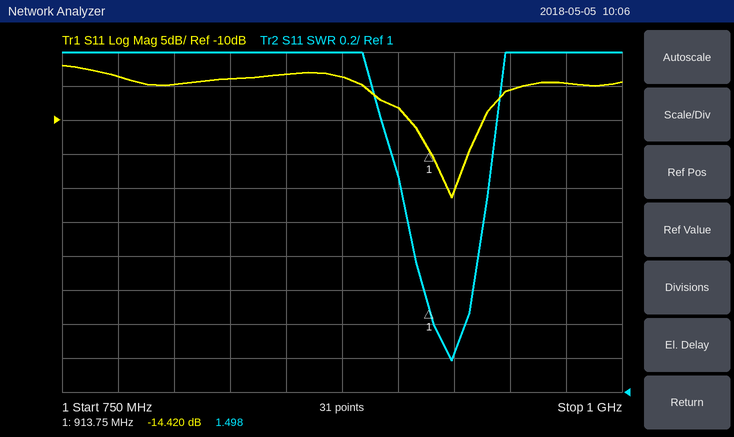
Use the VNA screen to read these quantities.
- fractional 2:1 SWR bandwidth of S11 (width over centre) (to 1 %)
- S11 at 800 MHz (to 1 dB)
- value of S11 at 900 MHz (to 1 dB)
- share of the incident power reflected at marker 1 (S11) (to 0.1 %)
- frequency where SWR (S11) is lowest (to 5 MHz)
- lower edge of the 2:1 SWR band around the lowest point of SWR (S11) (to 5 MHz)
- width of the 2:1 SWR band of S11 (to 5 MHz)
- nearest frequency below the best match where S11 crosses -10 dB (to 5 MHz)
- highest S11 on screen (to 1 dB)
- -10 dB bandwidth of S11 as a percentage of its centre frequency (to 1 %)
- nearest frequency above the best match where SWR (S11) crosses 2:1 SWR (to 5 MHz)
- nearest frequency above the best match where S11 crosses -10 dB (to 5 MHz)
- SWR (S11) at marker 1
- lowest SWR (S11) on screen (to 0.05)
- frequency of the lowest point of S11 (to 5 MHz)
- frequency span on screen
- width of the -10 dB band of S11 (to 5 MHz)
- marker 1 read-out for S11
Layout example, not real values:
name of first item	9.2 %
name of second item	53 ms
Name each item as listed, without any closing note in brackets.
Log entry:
fractional 2:1 SWR bandwidth of S11 (width over centre)	4 %
S11 at 800 MHz	-5 dB
value of S11 at 900 MHz	-8 dB
share of the incident power reflected at marker 1 (S11)	3.6 %
frequency where SWR (S11) is lowest	925 MHz
lower edge of the 2:1 SWR band around the lowest point of SWR (S11)	905 MHz
width of the 2:1 SWR band of S11	35 MHz
nearest frequency below the best match where S11 crosses -10 dB	905 MHz
highest S11 on screen	-2 dB
-10 dB bandwidth of S11 as a percentage of its centre frequency	4 %
nearest frequency above the best match where SWR (S11) crosses 2:1 SWR	940 MHz
nearest frequency above the best match where S11 crosses -10 dB	940 MHz
SWR (S11) at marker 1	1.498
lowest SWR (S11) on screen	1.20
frequency of the lowest point of S11	925 MHz
frequency span on screen	250 MHz
width of the -10 dB band of S11	35 MHz
marker 1 read-out for S11	-14.420 dB
